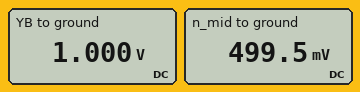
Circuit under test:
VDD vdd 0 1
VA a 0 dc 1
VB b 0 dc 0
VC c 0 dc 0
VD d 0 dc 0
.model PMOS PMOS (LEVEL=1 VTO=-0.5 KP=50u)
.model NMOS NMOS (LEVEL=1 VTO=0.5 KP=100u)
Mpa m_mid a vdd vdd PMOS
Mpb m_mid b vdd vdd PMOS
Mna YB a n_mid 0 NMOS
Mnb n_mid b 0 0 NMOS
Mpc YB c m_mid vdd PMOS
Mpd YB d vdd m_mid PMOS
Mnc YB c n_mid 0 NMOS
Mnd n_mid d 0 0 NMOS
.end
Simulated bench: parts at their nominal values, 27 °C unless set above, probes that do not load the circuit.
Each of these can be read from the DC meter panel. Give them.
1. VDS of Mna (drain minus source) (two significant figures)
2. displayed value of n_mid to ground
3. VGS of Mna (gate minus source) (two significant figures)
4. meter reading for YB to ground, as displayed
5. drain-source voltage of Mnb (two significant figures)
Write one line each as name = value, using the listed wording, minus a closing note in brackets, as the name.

VDS of Mna (drain minus source) = 500 mV
displayed value of n_mid to ground = 499.5 mV
VGS of Mna (gate minus source) = 500 mV
meter reading for YB to ground, as displayed = 1.000 V
drain-source voltage of Mnb = 500 mV
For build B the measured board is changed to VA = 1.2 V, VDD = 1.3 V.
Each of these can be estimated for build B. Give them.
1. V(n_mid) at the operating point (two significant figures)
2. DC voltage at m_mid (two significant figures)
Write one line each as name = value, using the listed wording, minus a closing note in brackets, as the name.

V(n_mid) at the operating point = 700 mV
DC voltage at m_mid = 1.3 V
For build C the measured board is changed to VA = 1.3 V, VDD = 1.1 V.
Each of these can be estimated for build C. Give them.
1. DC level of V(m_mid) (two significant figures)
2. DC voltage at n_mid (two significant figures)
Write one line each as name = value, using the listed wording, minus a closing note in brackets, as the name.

DC level of V(m_mid) = 1.1 V
DC voltage at n_mid = 800 mV
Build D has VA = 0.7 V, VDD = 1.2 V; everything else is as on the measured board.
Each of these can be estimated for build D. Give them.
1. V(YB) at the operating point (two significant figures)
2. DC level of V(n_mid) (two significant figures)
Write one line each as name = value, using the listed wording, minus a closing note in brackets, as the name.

V(YB) at the operating point = 1.2 V
DC level of V(n_mid) = 200 mV
